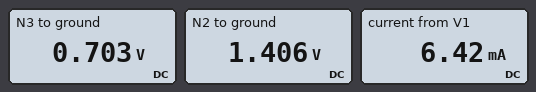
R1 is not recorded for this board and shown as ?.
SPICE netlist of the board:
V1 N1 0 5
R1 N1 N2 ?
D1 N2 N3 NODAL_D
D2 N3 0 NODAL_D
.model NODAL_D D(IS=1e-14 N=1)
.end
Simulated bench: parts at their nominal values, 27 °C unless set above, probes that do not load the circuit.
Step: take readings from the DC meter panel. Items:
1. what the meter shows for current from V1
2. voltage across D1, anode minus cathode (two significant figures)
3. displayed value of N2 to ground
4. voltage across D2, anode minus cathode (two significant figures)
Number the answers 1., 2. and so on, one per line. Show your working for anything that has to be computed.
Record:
1. 6.42 mA
2. 1.406 V - 703 mV = 700 mV
3. 1.406 V
4. 703 mV = 700 mV
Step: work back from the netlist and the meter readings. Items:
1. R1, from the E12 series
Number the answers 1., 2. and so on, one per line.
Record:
1. 560 Ω
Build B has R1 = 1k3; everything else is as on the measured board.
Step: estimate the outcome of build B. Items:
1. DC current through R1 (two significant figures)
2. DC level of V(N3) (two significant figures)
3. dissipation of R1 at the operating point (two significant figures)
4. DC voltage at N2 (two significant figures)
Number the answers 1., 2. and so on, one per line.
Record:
1. 2.8 mA
2. 680 mV
3. 10 mW
4. 1.4 V
